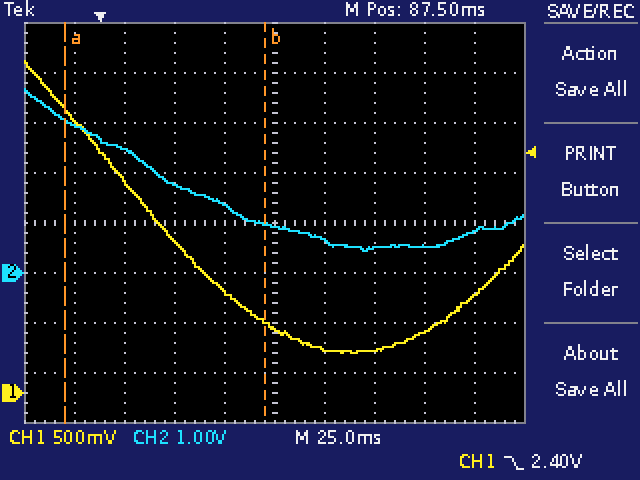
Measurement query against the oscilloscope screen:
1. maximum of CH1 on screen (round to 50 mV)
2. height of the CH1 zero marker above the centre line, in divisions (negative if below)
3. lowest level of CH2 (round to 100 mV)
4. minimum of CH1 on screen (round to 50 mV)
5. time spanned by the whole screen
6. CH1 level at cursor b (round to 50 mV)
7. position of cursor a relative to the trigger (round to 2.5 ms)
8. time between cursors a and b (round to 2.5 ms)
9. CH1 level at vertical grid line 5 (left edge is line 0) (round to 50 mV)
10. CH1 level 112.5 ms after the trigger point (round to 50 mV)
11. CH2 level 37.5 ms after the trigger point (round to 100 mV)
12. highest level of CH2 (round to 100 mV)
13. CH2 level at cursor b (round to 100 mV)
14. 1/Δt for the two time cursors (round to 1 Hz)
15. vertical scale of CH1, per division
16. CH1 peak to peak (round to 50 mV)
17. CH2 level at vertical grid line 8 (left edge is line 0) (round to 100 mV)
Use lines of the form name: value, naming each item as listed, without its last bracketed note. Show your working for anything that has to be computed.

maximum of CH1 on screen: 3.30 V
height of the CH1 zero marker above the centre line, in divisions: -3.4 div
lowest level of CH2: 400 mV
minimum of CH1 on screen: 400 mV
time spanned by the whole screen: 250 ms
CH1 level at cursor b: 700 mV
position of cursor a relative to the trigger: -17.5 ms
time between cursors a and b: 100.0 ms
CH1 level at vertical grid line 5 (left edge is line 0): 650 mV
CH1 level 112.5 ms after the trigger point: 450 mV
CH2 level 37.5 ms after the trigger point: 1.8 V
highest level of CH2: 3.7 V
CH2 level at cursor b: 1.0 V
1/Δt for the two time cursors: 1 / 100.0 ms ≈ 10 Hz
vertical scale of CH1, per division: 500 mV
CH1 peak to peak: 3.30 V − (400 mV) = 2.90 V
CH2 level at vertical grid line 8 (left edge is line 0): 500 mV
